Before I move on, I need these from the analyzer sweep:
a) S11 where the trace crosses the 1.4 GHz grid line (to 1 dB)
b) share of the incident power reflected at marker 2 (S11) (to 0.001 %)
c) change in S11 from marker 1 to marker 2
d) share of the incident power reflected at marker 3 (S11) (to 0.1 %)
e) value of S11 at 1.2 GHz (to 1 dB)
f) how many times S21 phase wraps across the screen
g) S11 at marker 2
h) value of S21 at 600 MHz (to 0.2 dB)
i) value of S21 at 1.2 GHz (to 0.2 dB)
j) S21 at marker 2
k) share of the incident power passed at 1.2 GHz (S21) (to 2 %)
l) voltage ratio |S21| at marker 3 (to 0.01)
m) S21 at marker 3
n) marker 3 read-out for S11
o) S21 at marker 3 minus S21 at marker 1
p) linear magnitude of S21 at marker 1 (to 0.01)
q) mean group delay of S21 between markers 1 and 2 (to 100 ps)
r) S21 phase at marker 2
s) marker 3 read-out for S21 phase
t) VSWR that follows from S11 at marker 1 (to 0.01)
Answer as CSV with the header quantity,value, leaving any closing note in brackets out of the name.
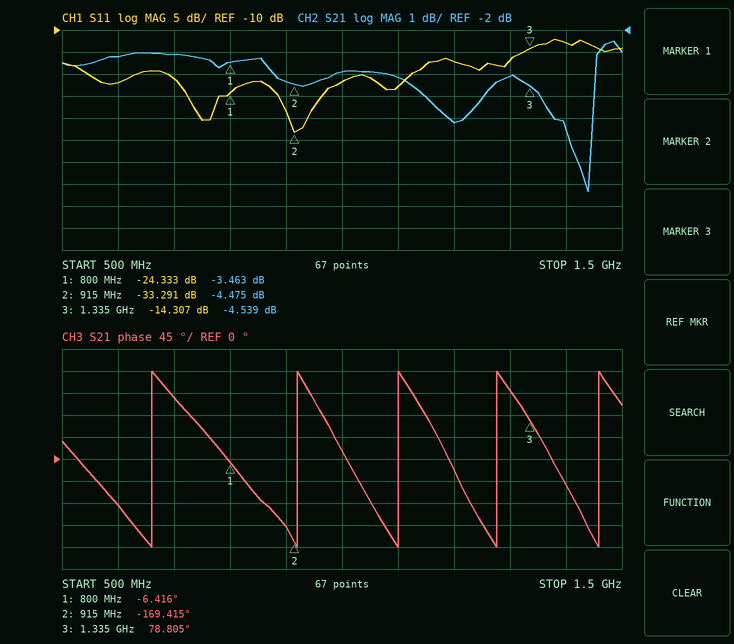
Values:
quantity,value
S11 where the trace crosses the 1.4 GHz grid line,-13 dB
share of the incident power reflected at marker 2 (S11),0.047 %
change in S11 from marker 1 to marker 2,-8.958 dB
share of the incident power reflected at marker 3 (S11),3.7 %
value of S11 at 1.2 GHz,-17 dB
how many times S21 phase wraps across the screen,5
S11 at marker 2,-33.291 dB
value of S21 at 600 MHz,-3.2 dB
value of S21 at 1.2 GHz,-6.2 dB
S21 at marker 2,-4.475 dB
share of the incident power passed at 1.2 GHz (S21),24 %
voltage ratio |S21| at marker 3,0.59
S21 at marker 3,-4.539 dB
marker 3 read-out for S11,-14.307 dB
S21 at marker 3 minus S21 at marker 1,-1.076 dB
linear magnitude of S21 at marker 1,0.67
mean group delay of S21 between markers 1 and 2,3.9 ns
S21 phase at marker 2,-169.415°
marker 3 read-out for S21 phase,78.805°
VSWR that follows from S11 at marker 1,1.13
